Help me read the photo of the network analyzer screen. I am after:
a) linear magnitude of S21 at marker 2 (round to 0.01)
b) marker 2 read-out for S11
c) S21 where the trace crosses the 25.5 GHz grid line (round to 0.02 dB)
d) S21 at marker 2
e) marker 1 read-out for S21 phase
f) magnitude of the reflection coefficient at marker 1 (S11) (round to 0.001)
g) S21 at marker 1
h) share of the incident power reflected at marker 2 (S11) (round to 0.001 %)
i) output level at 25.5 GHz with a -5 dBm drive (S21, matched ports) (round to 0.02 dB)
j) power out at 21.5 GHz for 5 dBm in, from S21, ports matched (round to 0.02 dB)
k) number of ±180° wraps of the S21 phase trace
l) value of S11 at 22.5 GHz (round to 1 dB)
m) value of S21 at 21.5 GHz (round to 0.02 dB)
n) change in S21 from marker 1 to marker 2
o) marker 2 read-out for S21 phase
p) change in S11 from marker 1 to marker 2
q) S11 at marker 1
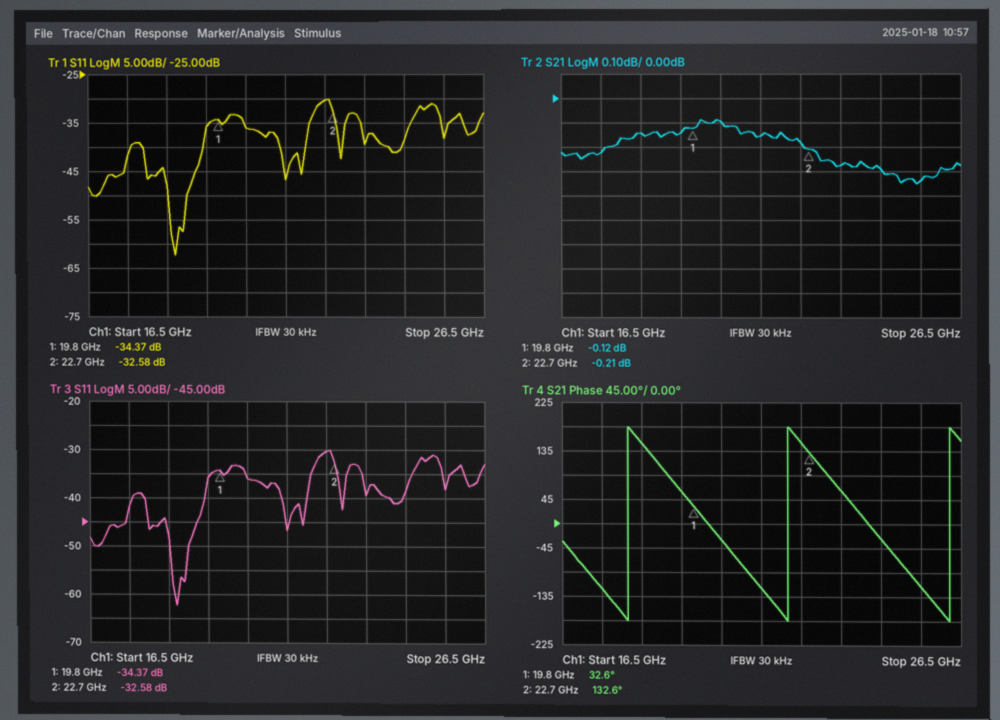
0.98
-32.58 dB
-0.34 dB
-0.21 dB
32.6°
0.019
-0.12 dB
0.055 %
-5.34 dBm
4.84 dBm
3
-30 dB
-0.16 dB
-0.09 dB
132.6°
1.79 dB
-34.37 dB
